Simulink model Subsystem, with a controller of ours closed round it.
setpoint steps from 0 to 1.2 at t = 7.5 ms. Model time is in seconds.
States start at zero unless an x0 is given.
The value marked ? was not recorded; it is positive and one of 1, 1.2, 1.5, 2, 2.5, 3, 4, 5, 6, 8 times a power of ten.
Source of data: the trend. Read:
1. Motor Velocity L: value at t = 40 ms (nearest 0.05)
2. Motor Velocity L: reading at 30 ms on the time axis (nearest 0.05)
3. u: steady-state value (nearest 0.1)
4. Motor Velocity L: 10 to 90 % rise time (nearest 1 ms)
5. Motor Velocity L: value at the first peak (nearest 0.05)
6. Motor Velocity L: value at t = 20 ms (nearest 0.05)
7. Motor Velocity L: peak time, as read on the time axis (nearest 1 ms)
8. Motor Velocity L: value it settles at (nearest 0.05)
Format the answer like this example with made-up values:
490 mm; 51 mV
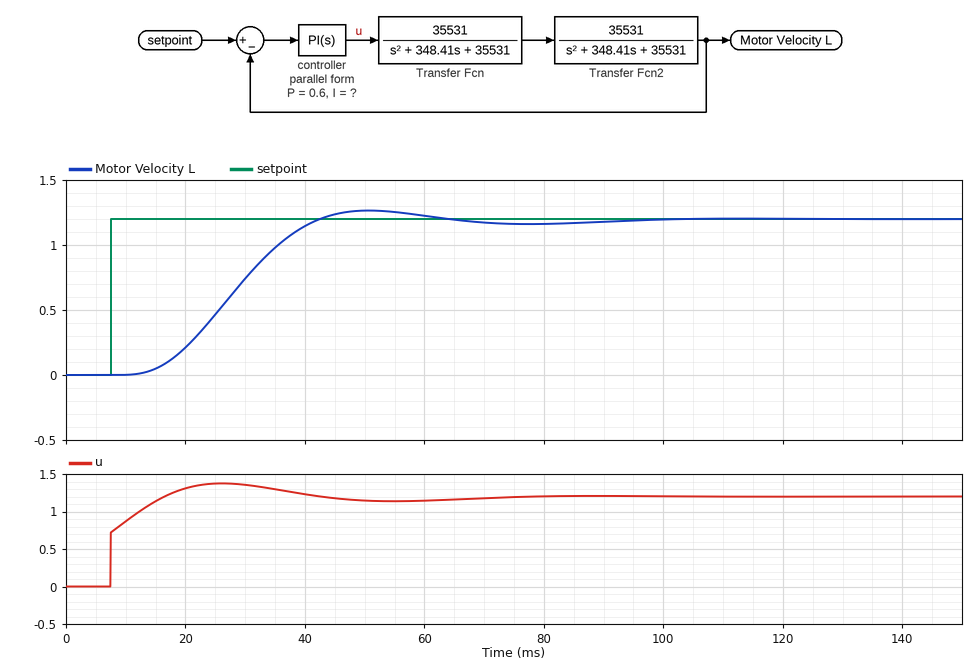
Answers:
1.15; 0.75; 1.2; 20 ms; 1.25; 0.20; 51 ms; 1.20
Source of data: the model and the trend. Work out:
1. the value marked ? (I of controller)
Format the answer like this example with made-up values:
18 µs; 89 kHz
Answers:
50
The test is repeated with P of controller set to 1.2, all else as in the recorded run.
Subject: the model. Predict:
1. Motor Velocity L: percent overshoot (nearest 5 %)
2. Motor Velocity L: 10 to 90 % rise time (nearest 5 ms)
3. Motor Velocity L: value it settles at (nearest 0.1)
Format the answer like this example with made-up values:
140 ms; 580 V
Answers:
10 %; 15 ms; 1.2
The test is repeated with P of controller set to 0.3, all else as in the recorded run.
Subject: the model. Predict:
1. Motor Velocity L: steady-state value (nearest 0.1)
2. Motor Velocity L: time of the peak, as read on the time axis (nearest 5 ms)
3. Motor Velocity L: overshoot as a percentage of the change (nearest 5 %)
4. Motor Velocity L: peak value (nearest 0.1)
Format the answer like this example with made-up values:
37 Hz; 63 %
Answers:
1.2; 60 ms; 15 %; 1.4
